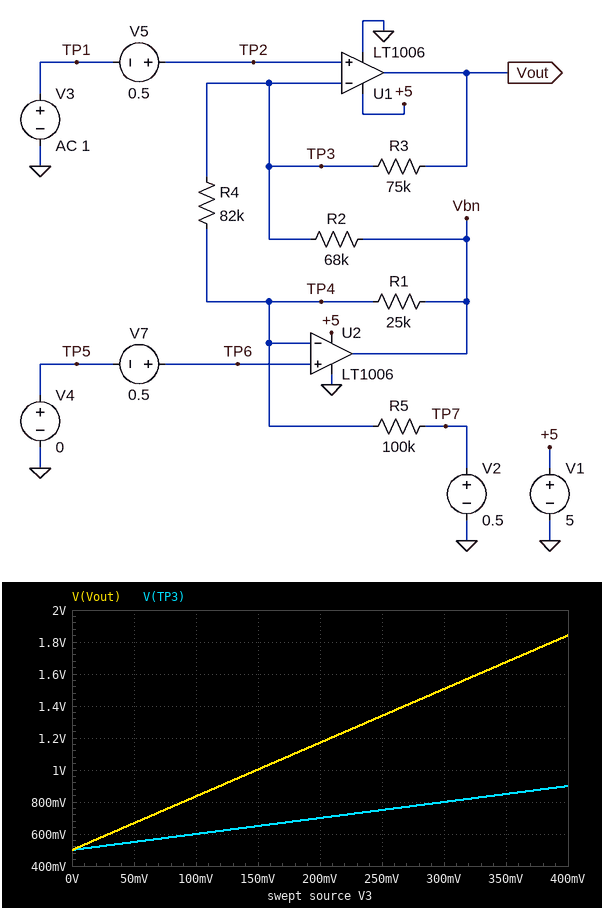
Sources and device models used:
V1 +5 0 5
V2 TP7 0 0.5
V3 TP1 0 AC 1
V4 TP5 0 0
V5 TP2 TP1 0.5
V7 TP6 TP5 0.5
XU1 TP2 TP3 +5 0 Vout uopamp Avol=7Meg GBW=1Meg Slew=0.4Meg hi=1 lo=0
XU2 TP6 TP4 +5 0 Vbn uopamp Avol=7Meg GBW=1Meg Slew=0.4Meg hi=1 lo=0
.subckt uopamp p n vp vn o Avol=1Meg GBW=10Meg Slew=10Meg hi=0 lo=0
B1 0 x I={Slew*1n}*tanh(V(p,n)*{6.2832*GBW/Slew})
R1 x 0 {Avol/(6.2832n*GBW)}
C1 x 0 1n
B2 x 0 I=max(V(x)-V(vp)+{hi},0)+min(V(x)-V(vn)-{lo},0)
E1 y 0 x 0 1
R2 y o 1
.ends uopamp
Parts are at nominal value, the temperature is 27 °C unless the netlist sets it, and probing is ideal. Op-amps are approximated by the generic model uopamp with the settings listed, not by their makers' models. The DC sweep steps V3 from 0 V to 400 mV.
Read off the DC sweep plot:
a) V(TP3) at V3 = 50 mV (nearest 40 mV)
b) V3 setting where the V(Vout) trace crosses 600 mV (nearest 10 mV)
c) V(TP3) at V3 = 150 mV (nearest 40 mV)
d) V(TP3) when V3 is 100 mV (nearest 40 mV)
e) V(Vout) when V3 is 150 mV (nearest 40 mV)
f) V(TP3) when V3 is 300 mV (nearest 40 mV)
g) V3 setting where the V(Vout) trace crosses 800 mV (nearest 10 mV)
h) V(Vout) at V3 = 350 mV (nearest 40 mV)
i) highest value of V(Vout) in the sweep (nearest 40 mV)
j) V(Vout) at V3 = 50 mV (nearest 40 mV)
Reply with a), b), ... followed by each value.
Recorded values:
a) 560 mV
b) 30 mV
c) 640 mV
d) 600 mV
e) 1.00 V
f) 800 mV
g) 90 mV
h) 1.68 V
i) 1.84 V
j) 680 mV
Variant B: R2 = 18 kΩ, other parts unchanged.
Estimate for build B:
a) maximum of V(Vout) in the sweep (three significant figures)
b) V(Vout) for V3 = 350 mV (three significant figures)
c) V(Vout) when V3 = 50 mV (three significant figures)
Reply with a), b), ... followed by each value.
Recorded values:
a) 3.44 V
b) 3.07 V
c) 868 mV
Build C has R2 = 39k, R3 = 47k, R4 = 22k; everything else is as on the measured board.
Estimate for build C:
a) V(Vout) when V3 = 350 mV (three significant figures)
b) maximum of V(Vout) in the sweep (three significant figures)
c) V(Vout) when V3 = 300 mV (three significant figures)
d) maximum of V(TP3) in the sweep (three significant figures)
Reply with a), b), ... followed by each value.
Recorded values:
a) 2.50 V
b) 2.78 V
c) 2.21 V
d) 900 mV
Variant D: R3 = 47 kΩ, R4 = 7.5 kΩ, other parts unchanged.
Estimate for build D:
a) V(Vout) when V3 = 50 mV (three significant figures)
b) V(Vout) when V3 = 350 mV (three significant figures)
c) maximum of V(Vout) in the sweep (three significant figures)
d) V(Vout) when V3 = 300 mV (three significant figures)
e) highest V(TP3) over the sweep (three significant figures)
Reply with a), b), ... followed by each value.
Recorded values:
a) 1.01 V
b) 2.72 V
c) 2.89 V
d) 2.55 V
e) 900 mV
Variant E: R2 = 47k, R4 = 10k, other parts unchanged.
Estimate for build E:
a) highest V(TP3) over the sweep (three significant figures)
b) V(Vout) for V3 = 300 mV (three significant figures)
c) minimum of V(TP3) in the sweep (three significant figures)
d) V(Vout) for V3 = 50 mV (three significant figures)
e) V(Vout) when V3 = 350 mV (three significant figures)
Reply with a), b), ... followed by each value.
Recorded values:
a) 834 mV
b) 3.83 V
c) 500 mV
d) 1.20 V
e) 4.00 V
